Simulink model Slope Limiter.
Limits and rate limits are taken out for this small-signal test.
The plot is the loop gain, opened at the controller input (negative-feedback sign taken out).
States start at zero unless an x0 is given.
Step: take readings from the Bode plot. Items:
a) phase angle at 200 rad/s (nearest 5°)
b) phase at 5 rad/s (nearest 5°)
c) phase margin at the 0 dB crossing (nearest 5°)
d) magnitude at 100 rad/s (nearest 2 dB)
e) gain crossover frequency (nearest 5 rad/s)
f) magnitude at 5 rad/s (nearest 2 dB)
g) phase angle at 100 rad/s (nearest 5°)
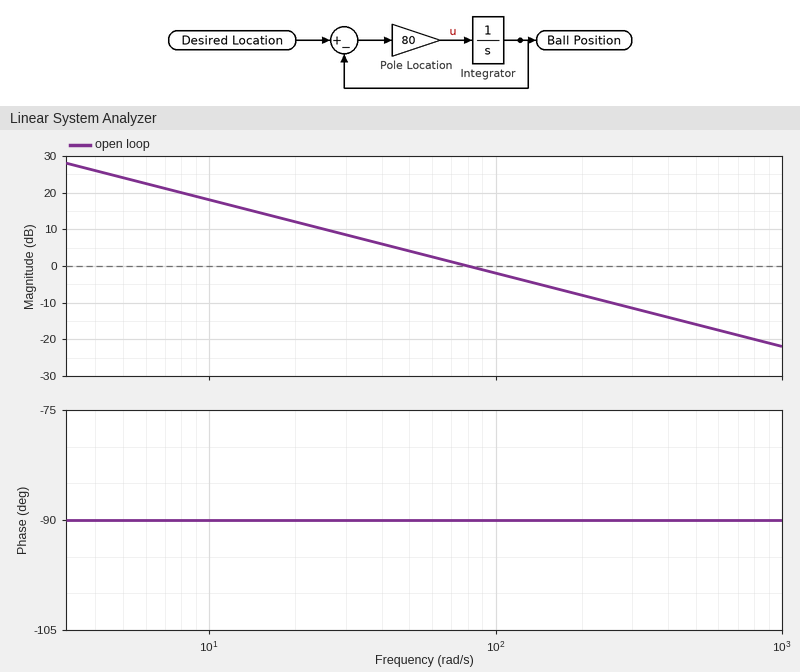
-90°
-90°
90°
-2 dB
80 rad/s
24 dB
-90°
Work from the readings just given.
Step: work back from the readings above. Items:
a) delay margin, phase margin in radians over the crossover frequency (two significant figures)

0.020 s
